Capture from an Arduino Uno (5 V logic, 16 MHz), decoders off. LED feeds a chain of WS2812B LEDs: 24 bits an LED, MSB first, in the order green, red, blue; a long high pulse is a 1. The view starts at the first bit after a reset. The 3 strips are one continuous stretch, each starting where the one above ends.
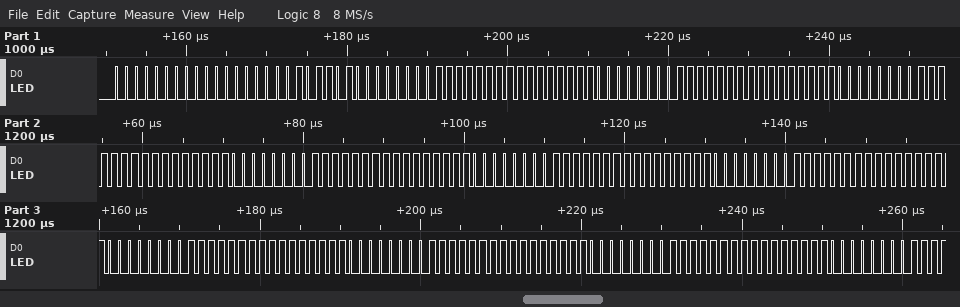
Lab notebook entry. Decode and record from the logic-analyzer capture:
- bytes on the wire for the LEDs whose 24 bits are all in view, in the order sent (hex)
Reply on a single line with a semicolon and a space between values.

00 00 2D 00 FF FF 00 FF FF 00 FF FF 00 FF FF 00 FF FF 00 FF FF 00 FF FF 00 FF FF 00 FF FF
